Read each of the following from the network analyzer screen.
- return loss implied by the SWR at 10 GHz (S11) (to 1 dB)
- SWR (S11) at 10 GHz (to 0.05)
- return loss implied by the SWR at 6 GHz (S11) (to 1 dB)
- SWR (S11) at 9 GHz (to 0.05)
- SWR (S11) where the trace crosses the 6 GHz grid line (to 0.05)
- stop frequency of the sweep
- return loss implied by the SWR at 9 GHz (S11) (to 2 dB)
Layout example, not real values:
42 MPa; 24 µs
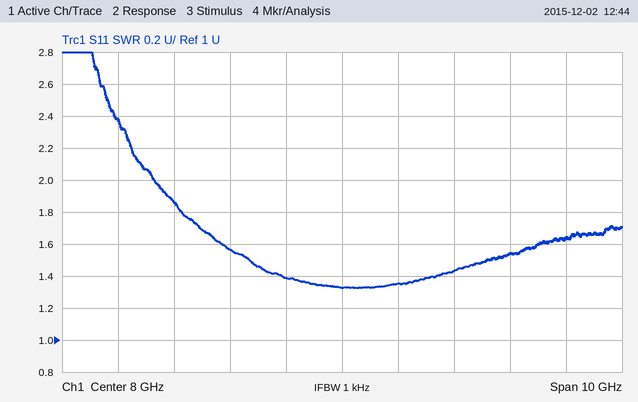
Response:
15 dB; 1.45; 13 dB; 1.35; 1.55; 13 GHz; 16 dB
